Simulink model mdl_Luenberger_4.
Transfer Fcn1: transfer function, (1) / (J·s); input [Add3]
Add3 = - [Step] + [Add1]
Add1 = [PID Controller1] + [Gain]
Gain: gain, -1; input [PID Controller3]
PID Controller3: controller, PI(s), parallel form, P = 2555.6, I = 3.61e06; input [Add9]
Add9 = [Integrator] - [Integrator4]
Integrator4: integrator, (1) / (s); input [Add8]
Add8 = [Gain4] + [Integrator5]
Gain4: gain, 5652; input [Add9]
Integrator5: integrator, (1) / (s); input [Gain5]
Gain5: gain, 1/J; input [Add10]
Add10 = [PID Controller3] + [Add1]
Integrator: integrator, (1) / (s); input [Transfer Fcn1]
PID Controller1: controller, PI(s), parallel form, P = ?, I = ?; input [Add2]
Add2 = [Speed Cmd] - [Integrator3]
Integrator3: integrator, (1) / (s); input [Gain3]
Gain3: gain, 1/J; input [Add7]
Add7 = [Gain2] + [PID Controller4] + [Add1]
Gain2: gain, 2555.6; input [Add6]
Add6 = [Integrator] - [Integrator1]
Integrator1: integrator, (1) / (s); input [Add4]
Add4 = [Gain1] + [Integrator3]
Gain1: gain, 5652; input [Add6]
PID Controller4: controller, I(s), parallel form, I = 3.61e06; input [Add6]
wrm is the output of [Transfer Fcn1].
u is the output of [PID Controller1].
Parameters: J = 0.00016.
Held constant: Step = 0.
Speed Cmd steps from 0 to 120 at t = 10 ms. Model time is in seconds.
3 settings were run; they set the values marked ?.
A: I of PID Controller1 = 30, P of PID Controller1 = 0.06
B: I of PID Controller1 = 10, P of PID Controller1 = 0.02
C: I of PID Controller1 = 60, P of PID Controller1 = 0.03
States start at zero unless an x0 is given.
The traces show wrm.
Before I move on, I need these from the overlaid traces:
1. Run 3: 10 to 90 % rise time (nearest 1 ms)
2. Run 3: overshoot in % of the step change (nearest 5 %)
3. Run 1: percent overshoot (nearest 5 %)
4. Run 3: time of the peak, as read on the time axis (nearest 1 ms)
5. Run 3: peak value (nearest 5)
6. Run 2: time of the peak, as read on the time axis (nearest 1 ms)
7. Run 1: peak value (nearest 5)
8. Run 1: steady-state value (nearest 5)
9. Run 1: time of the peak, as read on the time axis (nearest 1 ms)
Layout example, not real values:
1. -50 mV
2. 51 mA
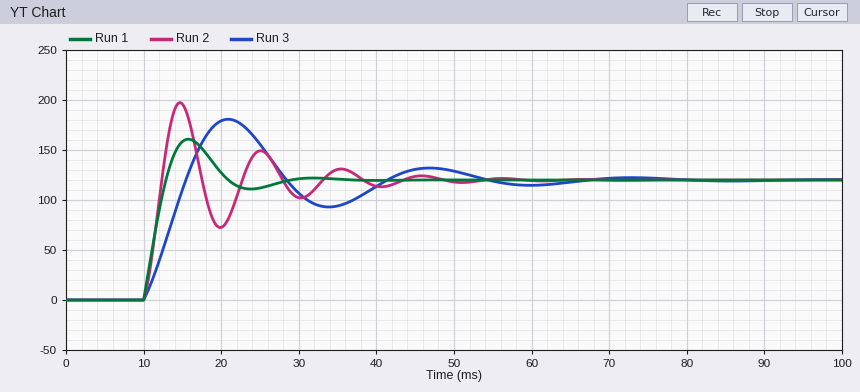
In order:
1. 4 ms
2. 50 %
3. 35 %
4. 21 ms
5. 180
6. 15 ms
7. 160
8. 120
9. 16 ms
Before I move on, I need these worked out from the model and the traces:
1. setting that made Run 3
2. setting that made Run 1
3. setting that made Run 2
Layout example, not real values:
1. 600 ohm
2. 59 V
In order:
1. B
2. A
3. C
